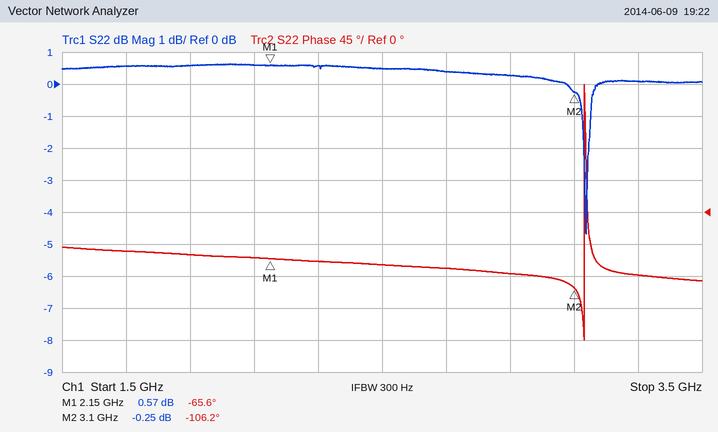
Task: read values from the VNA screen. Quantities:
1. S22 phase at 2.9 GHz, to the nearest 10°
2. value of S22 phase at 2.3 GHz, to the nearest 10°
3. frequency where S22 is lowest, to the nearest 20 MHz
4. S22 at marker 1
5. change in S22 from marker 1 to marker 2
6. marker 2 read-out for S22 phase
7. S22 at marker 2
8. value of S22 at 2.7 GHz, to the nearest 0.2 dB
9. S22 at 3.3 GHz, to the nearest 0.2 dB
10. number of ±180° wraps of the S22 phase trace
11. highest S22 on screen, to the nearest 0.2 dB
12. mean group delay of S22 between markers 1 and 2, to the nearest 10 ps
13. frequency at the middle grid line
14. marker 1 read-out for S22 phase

-90°
-70°
3.14 GHz
0.57 dB
-0.82 dB
-106.2°
-0.25 dB
0.4 dB
0.0 dB
1
0.6 dB
120 ps
2.5 GHz
-65.6°
